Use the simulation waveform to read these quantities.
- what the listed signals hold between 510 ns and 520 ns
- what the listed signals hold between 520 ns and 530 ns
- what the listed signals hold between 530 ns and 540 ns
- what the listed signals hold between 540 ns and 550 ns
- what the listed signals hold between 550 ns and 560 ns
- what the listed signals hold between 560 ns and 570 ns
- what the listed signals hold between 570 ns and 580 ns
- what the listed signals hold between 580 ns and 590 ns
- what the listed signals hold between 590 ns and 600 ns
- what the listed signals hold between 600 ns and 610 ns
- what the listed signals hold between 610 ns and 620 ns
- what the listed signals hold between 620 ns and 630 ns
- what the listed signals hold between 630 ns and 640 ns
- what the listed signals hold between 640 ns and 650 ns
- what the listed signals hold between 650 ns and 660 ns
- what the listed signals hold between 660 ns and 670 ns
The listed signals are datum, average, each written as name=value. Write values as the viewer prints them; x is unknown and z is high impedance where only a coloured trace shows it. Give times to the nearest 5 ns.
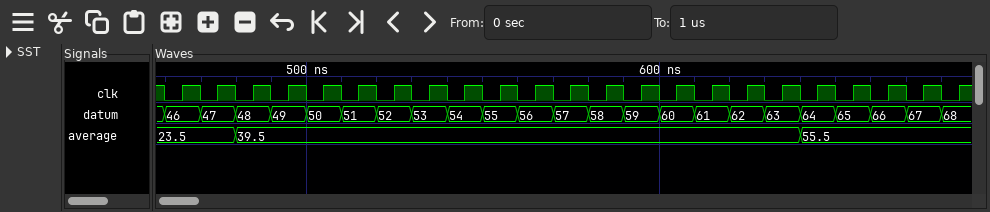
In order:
datum=51, average=39.5
datum=52, average=39.5
datum=53, average=39.5
datum=54, average=39.5
datum=55, average=39.5
datum=56, average=39.5
datum=57, average=39.5
datum=58, average=39.5
datum=59, average=39.5
datum=60, average=39.5
datum=61, average=39.5
datum=62, average=39.5
datum=63, average=39.5
datum=64, average=55.5
datum=65, average=55.5
datum=66, average=55.5
